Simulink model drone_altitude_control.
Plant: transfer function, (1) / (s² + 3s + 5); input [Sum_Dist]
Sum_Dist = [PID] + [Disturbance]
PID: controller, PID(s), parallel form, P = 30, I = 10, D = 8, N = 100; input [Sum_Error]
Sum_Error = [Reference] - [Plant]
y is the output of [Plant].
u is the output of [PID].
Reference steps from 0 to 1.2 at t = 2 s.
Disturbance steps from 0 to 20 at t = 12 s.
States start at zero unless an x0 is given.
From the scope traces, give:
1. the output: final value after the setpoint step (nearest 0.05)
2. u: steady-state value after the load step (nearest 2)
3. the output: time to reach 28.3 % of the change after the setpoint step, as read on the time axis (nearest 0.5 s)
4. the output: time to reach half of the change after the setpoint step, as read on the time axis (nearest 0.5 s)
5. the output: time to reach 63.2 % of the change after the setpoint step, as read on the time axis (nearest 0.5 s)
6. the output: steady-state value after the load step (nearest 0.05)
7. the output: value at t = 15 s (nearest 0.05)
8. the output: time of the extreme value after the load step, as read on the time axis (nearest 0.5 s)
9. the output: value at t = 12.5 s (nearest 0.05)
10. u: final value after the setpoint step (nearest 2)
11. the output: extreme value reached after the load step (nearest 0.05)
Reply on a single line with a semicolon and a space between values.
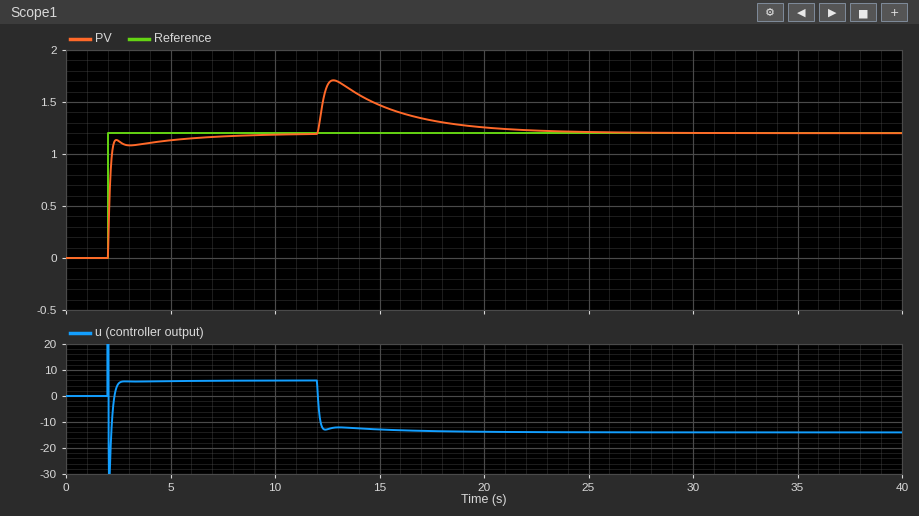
1.20; -14; 2.0 s; 2.0 s; 2.0 s; 1.20; 1.45; 13.0 s; 1.65; 6; 1.70
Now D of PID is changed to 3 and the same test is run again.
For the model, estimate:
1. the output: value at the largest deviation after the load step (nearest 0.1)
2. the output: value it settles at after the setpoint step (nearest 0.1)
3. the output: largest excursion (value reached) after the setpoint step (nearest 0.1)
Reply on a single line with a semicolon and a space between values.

1.8; 1.2; 1.3
